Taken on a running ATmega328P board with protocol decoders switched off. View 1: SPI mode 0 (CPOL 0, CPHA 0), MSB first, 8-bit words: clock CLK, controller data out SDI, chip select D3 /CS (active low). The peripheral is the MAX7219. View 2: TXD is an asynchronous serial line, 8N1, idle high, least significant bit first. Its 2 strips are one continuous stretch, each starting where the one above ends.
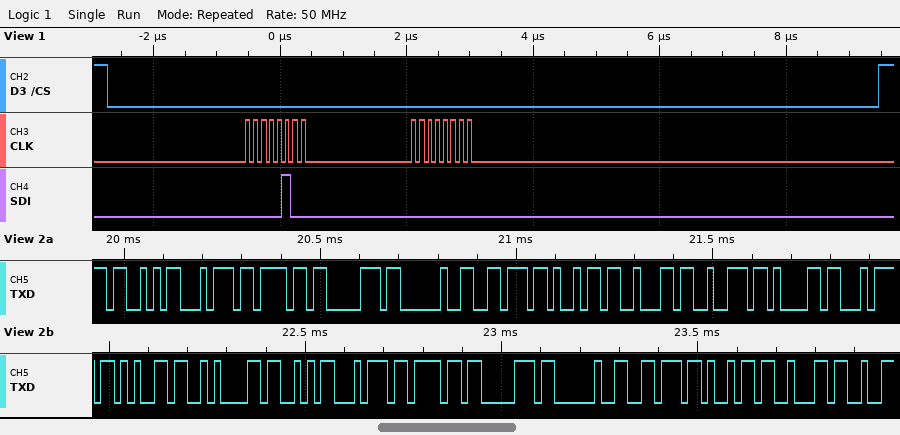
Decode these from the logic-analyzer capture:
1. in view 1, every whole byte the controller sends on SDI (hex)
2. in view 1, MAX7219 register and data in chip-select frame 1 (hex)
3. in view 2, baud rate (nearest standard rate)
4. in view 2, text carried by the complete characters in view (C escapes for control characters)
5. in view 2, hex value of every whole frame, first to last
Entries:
04 00
register 0x4, data 0x00
57600 baud
"Stop vibrate\nStop vib"
0x53 0x74 0x6F 0x70 0x20 0x76 0x69 0x62 0x72 0x61 0x74 0x65 0x0A 0x53 0x74 0x6F 0x70 0x20 0x76 0x69 0x62
